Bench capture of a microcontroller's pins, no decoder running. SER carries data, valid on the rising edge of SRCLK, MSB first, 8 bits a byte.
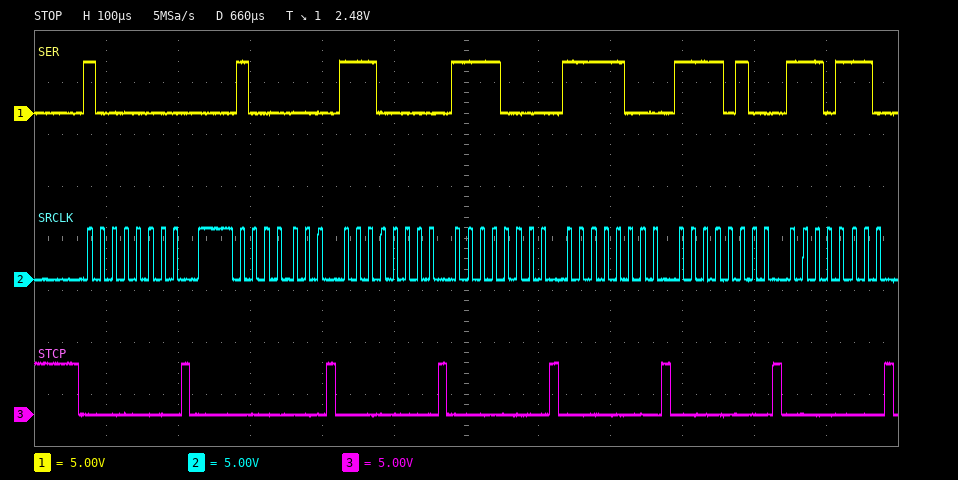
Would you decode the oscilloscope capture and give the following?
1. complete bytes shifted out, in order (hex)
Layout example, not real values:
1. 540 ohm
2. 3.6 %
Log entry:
1. 80 40 E0 F0 F8 F4 EE
